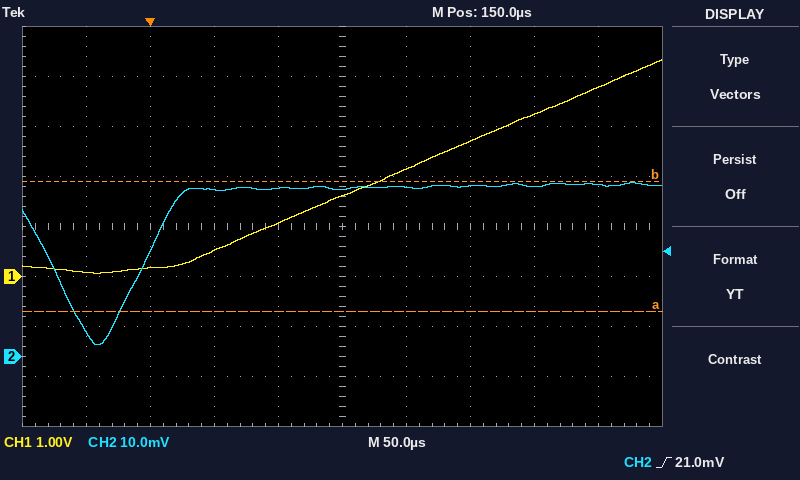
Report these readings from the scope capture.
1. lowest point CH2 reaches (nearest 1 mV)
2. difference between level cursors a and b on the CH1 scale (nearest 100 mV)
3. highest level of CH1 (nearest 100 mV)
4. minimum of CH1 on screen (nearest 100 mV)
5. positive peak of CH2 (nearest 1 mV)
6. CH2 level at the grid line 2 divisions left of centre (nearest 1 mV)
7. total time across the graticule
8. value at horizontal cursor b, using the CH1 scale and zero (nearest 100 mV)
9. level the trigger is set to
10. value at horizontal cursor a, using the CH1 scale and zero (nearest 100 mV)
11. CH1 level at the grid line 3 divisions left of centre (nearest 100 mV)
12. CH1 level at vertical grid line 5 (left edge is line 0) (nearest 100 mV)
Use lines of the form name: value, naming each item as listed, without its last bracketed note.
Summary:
lowest point CH2 reaches: 2 mV
difference between level cursors a and b on the CH1 scale: 2.6 V
highest level of CH1: 4.3 V
minimum of CH1 on screen: 100 mV
positive peak of CH2: 35 mV
CH2 level at the grid line 2 divisions left of centre: 33 mV
total time across the graticule: 500 µs
value at horizontal cursor b, using the CH1 scale and zero: 1.9 V
level the trigger is set to: 21.0 mV
value at horizontal cursor a, using the CH1 scale and zero: -700 mV
CH1 level at the grid line 3 divisions left of centre: 200 mV
CH1 level at vertical grid line 5 (left edge is line 0): 1.6 V
